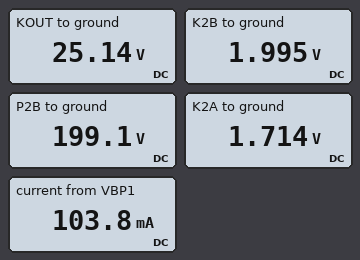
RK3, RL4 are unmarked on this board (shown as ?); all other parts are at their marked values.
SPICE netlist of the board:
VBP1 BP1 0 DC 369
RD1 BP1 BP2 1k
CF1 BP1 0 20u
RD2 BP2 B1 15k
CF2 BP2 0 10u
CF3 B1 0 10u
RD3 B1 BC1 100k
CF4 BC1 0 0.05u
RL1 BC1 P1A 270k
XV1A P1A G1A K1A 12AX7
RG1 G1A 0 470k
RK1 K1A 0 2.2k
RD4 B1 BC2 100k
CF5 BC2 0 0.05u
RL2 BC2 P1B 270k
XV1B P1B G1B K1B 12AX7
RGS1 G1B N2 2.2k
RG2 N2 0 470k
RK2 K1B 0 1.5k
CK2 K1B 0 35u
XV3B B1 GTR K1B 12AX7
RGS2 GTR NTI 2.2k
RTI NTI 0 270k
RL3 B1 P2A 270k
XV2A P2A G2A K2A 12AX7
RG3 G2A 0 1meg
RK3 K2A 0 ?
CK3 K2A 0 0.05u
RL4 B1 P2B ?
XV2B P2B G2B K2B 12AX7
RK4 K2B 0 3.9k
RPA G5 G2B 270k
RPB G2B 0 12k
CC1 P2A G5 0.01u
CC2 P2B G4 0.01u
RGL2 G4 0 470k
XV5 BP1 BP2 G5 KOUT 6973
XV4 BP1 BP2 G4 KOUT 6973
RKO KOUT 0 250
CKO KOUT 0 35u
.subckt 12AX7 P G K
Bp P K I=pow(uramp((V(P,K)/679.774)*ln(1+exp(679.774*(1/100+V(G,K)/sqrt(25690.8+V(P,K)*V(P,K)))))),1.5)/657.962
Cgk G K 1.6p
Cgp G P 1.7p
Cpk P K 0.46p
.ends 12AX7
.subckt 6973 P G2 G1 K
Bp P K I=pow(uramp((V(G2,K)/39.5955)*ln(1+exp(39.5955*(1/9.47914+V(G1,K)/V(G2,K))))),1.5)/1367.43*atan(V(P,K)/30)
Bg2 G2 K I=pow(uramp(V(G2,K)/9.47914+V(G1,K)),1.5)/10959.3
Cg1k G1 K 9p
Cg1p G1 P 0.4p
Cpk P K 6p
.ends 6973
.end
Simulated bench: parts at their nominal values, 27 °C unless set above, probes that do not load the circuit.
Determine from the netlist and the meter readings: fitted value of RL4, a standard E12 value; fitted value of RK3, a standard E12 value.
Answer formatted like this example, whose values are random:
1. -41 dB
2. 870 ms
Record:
1. 220 kΩ
2. 3.3 kΩ
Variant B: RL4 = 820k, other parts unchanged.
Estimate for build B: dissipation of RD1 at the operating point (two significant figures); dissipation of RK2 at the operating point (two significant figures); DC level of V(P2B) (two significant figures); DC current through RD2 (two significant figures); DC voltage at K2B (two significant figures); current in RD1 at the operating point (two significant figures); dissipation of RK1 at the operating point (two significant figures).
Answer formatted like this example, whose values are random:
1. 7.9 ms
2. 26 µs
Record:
1. 80 mW
2. 4.2 mW
3. 83 V
4. 3.0 mA
5. 1.1 V
6. 8.9 mA
7. 620 µW
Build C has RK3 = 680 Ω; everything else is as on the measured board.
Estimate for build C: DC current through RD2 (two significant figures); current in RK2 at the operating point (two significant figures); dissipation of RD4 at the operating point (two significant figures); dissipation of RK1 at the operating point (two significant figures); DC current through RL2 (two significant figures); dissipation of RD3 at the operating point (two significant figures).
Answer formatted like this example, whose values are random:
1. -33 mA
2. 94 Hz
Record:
1. 3.5 mA
2. 1.6 mA
3. 6.5 mW
4. 590 µW
5. 250 µA
6. 27 mW
